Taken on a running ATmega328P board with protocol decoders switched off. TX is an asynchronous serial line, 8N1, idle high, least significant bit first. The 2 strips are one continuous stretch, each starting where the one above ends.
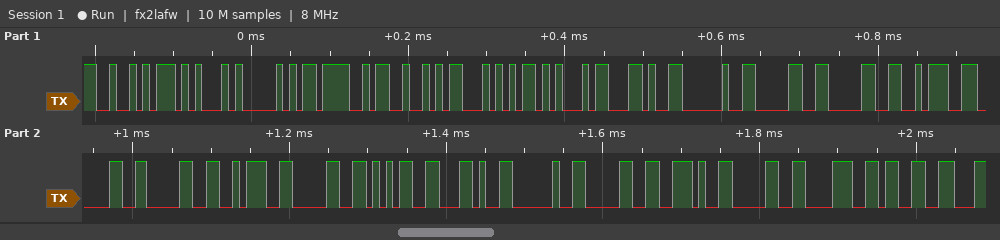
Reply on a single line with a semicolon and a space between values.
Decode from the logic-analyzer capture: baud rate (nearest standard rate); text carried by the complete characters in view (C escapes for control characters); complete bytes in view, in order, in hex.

115200 baud; "REPORTE, 00:00:05, 0.083"; 52 45 50 4F 52 54 45 2C 20 30 30 3A 30 30 3A 30 35 2C 20 30 2E 30 38 33
